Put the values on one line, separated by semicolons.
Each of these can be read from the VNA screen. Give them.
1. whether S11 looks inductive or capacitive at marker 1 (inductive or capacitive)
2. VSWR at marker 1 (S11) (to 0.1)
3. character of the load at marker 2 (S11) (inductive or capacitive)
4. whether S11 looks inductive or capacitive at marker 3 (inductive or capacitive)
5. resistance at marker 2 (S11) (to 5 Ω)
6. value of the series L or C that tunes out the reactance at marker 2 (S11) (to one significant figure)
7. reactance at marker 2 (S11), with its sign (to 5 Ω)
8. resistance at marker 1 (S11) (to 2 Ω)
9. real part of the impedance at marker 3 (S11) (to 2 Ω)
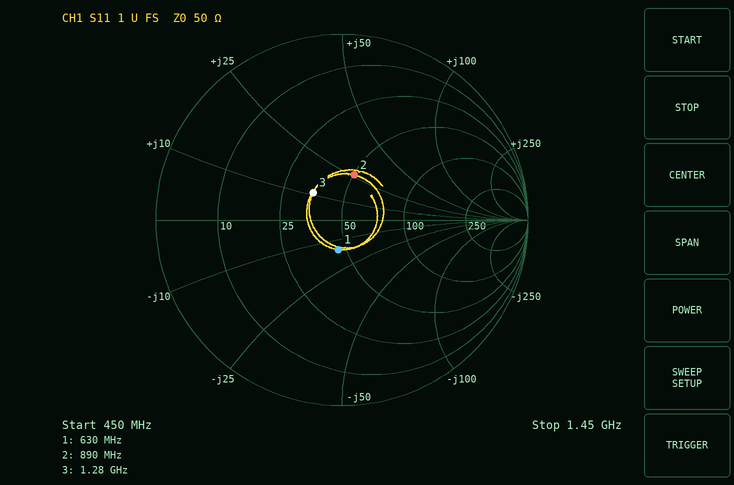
capacitive; 1.4; inductive; inductive; 50 Ω; 7 pF; +25 Ω; 46 Ω; 36 Ω
